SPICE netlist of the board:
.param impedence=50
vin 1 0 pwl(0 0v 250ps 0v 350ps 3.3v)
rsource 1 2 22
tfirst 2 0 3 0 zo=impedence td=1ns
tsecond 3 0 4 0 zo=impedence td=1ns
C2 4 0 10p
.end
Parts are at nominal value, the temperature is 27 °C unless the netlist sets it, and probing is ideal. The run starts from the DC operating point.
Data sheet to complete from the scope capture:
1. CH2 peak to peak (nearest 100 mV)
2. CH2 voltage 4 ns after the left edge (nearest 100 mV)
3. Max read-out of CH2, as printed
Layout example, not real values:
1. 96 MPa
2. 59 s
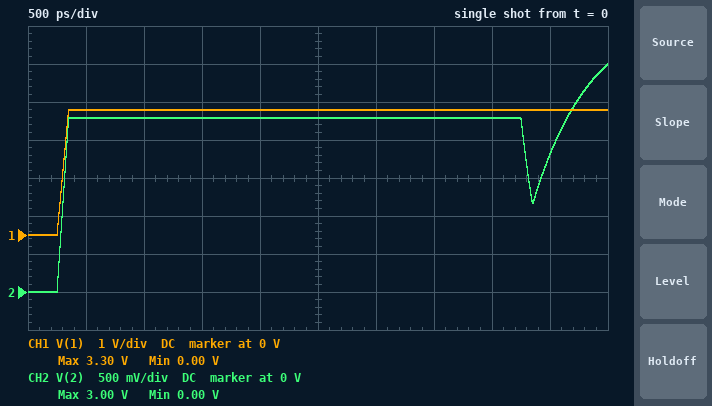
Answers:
1. 3.0 V
2. 2.3 V
3. 3.00 V
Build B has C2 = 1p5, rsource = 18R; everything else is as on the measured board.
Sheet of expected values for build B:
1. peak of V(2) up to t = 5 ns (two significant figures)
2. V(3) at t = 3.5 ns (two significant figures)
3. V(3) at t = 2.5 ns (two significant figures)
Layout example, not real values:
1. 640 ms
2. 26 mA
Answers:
1. 3.7 V
2. 4.5 V
3. 2.4 V
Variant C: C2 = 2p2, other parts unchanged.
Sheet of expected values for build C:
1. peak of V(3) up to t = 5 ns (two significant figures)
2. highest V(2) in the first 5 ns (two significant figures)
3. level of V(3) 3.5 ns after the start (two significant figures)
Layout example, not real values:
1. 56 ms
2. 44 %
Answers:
1. 4.6 V
2. 3.7 V
3. 3.8 V
